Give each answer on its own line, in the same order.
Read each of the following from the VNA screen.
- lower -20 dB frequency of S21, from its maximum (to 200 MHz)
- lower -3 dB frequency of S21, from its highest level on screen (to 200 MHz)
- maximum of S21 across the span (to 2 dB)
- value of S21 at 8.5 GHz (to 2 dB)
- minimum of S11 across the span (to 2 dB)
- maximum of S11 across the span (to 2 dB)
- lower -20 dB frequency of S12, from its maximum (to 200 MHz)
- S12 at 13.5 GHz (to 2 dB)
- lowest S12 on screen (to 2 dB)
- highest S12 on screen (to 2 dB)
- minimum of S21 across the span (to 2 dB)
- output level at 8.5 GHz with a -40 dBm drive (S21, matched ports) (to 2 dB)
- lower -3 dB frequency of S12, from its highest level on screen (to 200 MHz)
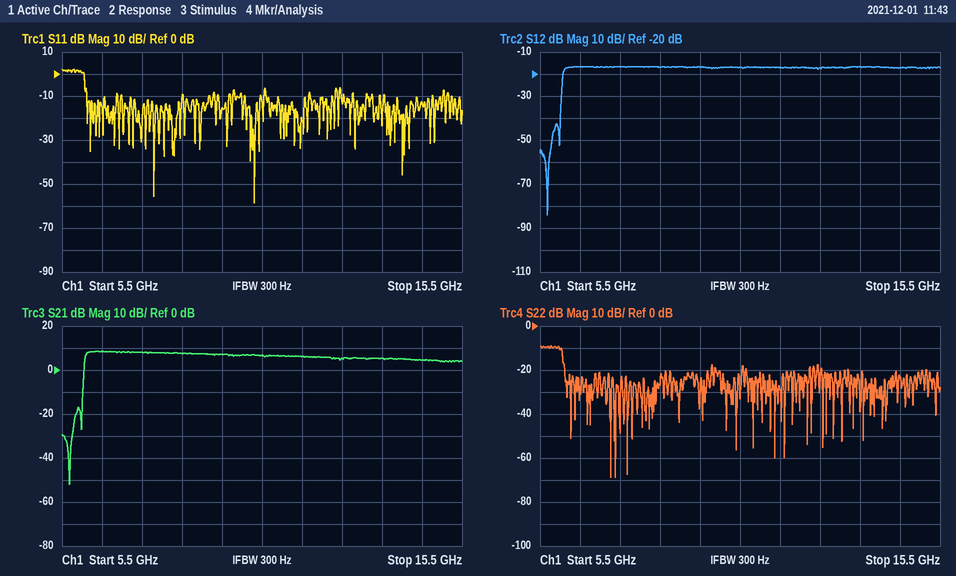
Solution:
6.0 GHz
6.0 GHz
8 dB
8 dB
-58 dB
2 dB
6.0 GHz
-16 dB
-84 dB
-16 dB
-52 dB
-32 dBm
6.0 GHz
